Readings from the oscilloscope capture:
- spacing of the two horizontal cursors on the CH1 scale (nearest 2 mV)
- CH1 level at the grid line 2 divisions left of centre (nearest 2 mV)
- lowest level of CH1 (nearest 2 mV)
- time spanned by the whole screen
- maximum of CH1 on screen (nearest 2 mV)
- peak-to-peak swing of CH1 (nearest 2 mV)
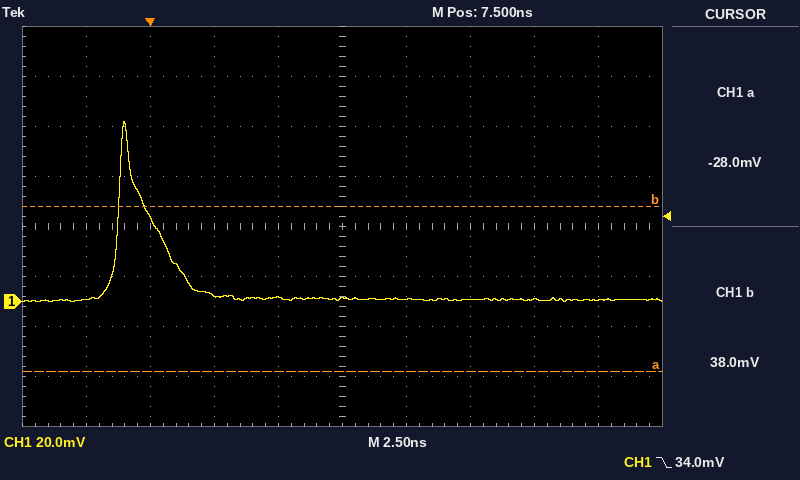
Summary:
66 mV
2 mV
0 mV
25 ns
72 mV
72 mV
